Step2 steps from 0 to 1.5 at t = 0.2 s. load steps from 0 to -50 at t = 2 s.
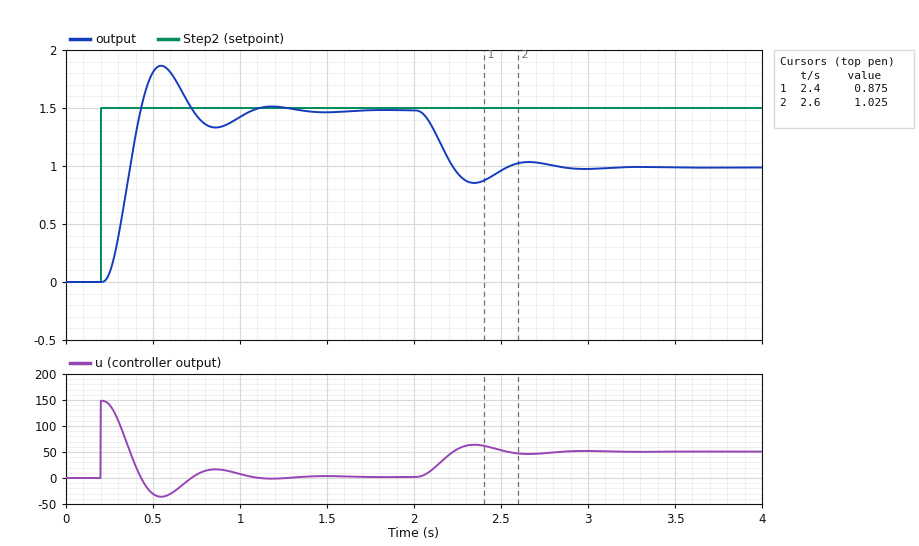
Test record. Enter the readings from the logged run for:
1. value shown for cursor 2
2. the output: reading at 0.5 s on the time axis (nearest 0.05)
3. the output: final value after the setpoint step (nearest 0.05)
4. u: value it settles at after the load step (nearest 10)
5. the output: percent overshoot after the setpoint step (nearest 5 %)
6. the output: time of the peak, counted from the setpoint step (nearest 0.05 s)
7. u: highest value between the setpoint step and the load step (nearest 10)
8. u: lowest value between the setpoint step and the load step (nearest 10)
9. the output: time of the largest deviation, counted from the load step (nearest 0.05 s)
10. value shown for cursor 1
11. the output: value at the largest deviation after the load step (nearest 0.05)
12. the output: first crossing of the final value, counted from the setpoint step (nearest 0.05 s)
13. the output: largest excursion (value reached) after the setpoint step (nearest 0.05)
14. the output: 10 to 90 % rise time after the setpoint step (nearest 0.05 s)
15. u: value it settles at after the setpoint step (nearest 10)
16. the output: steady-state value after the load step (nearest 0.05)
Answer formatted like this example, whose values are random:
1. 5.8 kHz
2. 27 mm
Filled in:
1. 1.025
2. 1.80
3. 1.50
4. 50
5. 25 %
6. 0.35 s
7. 150
8. -40
9. 0.35 s
10. 0.875
11. 0.85
12. 0.25 s
13. 1.85
14. 0.15 s
15. 0
16. 1.00
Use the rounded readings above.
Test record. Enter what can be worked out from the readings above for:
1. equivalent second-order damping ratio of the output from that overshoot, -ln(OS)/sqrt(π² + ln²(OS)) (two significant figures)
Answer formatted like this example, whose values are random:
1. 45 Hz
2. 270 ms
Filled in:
1. 0.40
